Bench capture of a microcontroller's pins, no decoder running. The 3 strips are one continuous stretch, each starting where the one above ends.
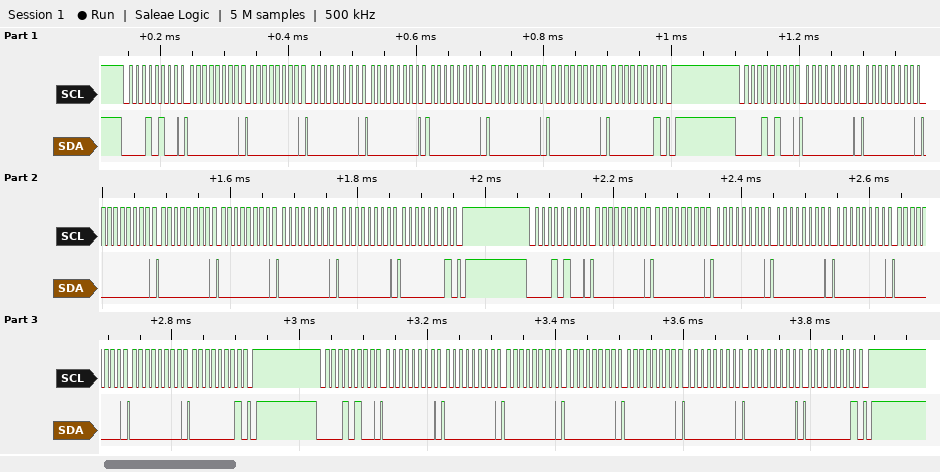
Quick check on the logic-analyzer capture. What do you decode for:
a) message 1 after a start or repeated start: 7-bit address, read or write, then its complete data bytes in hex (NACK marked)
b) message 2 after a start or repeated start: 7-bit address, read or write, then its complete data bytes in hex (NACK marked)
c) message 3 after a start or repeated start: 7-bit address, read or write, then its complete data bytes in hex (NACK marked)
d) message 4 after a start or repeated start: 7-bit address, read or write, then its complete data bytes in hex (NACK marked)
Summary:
0x0A write: 00 00 00 00 00 00 00 01
0x0A write: 00 00 00 00 00 00 00 01
0x0A write: 00 00 00 00 00 00 00 01
0x0A write: 00 00 00 00 00 00 00 01
